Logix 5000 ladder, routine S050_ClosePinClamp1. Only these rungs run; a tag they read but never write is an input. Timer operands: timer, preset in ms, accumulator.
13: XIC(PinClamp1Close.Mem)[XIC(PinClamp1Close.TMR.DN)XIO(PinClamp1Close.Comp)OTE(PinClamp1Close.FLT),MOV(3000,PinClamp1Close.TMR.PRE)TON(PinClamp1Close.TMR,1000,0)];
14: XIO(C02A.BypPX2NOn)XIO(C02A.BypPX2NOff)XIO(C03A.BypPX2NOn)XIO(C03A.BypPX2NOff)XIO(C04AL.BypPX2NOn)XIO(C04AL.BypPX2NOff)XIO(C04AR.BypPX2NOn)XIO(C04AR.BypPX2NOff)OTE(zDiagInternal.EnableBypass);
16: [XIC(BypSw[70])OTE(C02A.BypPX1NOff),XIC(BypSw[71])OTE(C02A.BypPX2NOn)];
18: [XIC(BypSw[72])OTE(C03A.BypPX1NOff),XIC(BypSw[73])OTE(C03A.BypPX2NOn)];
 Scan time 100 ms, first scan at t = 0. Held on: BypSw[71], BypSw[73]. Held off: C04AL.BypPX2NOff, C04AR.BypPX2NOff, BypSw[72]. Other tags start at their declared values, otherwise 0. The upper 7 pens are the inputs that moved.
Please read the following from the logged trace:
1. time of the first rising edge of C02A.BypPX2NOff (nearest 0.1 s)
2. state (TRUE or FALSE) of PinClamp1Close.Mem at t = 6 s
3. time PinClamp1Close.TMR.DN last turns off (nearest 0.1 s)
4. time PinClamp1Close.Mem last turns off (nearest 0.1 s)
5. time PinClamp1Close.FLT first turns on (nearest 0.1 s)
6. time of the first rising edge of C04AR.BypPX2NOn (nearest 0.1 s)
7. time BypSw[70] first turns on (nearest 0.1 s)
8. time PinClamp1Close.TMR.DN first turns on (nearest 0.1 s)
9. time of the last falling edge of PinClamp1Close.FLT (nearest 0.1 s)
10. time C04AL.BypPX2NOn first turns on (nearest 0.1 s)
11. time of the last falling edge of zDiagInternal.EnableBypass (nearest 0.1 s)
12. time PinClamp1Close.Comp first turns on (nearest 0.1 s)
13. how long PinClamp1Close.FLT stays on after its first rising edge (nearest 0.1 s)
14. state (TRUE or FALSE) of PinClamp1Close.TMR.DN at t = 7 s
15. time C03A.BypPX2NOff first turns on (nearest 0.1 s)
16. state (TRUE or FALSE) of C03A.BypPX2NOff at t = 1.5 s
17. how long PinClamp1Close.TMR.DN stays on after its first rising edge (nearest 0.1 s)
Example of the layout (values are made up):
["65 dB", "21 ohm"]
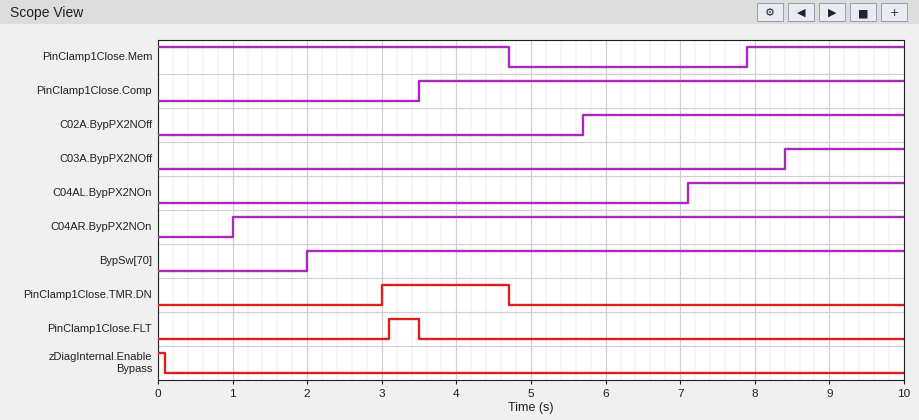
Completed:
["5.7 s", "FALSE", "4.7 s", "4.7 s", "3.1 s", "1.0 s", "2.0 s", "3.0 s", "3.5 s", "7.1 s", "0.1 s", "3.5 s", "0.4 s", "FALSE", "8.4 s", "FALSE", "1.7 s"]
